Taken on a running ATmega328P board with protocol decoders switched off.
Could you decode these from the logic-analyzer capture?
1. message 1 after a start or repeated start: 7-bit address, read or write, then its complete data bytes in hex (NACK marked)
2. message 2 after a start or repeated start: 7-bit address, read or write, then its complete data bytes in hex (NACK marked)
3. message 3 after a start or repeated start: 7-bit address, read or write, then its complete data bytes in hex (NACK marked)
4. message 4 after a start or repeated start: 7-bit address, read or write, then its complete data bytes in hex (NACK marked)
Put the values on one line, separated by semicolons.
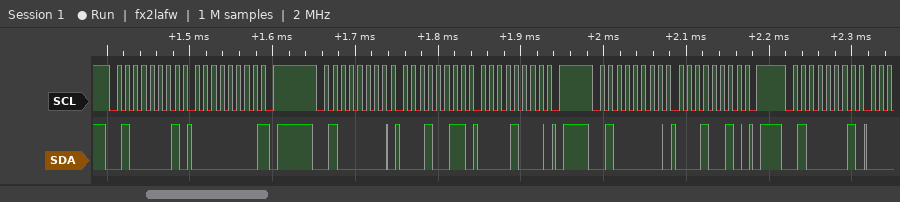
0x20 read: 00 NACK; 0x20 write: 13 08; 0x20 write: 12; 0x20 read
